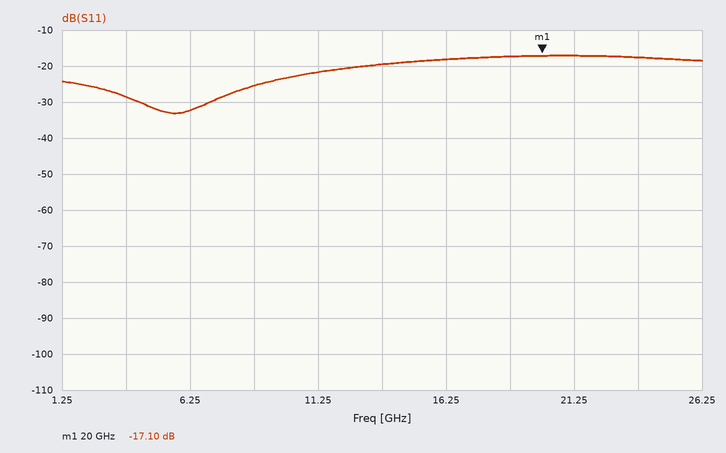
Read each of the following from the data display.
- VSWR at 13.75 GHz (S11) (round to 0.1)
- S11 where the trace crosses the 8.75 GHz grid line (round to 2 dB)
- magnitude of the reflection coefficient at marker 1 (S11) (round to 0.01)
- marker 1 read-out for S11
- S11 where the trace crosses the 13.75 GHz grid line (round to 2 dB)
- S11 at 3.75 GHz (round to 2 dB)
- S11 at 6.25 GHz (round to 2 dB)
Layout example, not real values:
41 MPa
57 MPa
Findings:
1.2
-26 dB
0.14
-17.10 dB
-20 dB
-28 dB
-32 dB
